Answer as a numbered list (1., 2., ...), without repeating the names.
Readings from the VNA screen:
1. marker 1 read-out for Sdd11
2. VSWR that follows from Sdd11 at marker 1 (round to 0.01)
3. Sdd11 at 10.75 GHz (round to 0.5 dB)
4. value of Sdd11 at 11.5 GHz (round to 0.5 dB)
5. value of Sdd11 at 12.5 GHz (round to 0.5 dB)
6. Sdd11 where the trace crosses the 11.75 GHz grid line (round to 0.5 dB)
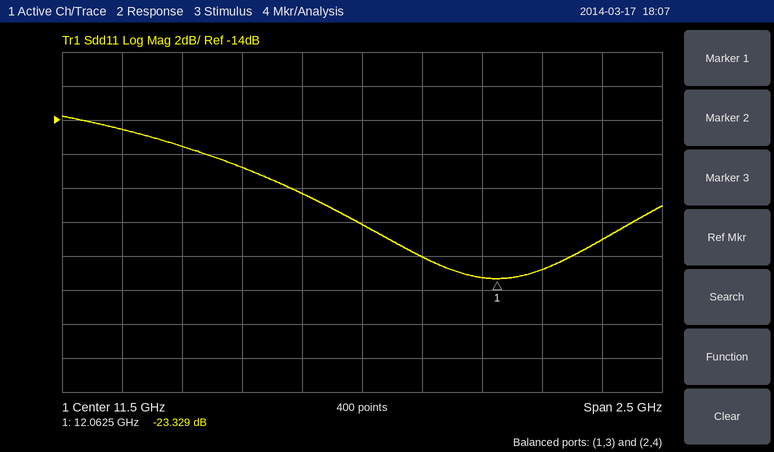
1. -23.329 dB
2. 1.15
3. -15.5 dB
4. -20.0 dB
5. -21.0 dB
6. -22.0 dB
